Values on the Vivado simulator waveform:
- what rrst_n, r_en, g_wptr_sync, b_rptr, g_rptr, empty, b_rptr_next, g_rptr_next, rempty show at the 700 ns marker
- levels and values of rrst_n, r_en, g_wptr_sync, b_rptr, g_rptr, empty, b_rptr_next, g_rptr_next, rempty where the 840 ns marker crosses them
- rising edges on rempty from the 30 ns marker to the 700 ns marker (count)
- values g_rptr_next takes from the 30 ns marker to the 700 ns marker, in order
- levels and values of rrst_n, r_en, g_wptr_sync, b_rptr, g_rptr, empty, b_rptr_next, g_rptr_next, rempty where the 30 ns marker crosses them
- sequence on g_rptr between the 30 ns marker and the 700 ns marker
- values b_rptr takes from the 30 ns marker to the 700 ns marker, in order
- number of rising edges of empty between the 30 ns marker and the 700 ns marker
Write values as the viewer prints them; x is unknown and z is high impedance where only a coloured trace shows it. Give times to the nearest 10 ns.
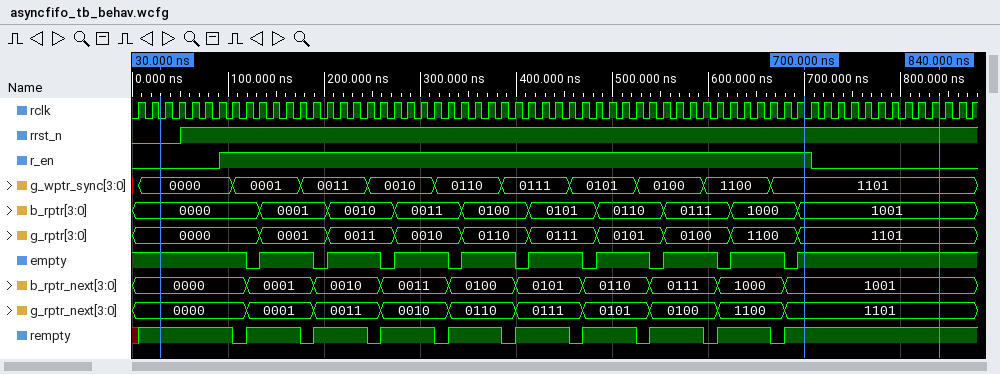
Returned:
rrst_n=1, r_en=1, g_wptr_sync=1101, b_rptr=1001, g_rptr=1101, empty=1, b_rptr_next=1001, g_rptr_next=1101, rempty=1
rrst_n=1, r_en=0, g_wptr_sync=1101, b_rptr=1001, g_rptr=1101, empty=1, b_rptr_next=1001, g_rptr_next=1101, rempty=1
9
0000, 0001, 0011, 0010, 0110, 0111, 0101, 0100, 1100, 1101
rrst_n=0, r_en=0, g_wptr_sync=0000, b_rptr=0000, g_rptr=0000, empty=1, b_rptr_next=0000, g_rptr_next=0000, rempty=1
0000, 0001, 0011, 0010, 0110, 0111, 0101, 0100, 1100, 1101
0000, 0001, 0010, 0011, 0100, 0101, 0110, 0111, 1000, 1001
9
